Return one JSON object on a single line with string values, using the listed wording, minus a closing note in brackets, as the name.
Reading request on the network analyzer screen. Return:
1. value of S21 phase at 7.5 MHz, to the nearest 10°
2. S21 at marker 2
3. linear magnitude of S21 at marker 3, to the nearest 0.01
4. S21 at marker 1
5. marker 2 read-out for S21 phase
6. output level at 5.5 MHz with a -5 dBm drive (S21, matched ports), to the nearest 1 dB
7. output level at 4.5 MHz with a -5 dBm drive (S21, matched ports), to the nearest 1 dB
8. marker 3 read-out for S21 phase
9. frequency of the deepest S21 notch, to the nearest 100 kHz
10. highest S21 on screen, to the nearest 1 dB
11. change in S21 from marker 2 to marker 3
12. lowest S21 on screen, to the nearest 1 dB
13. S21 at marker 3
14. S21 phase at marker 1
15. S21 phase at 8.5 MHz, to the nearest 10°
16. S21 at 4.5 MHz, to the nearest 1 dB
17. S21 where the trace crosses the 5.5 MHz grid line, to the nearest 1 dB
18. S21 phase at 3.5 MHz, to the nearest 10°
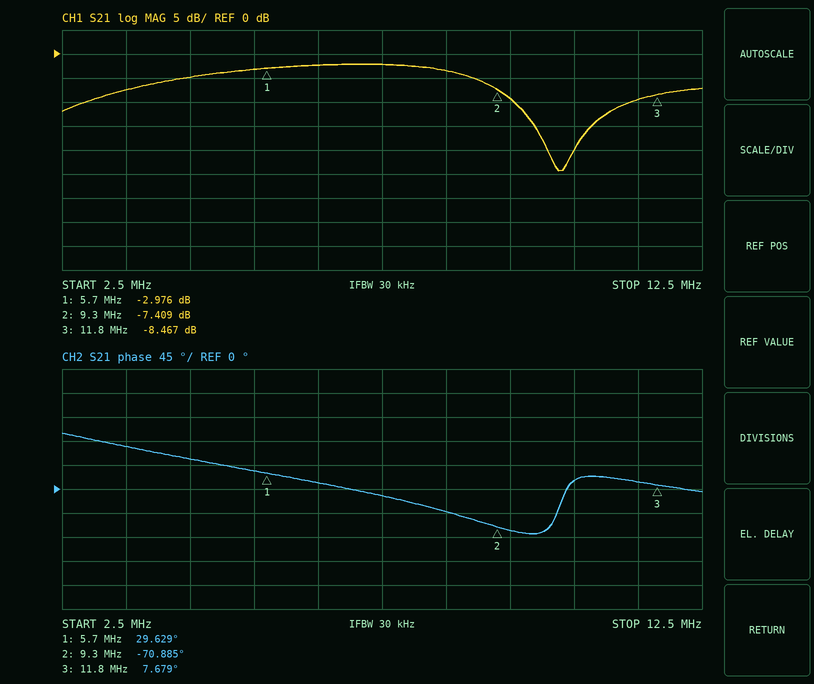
{"value of S21 phase at 7.5 MHz, to the nearest 10°": "-10°", "S21 at marker 2": "-7.409 dB", "linear magnitude of S21 at marker 3, to the nearest 0.01": "0.38", "S21 at marker 1": "-2.976 dB", "marker 2 read-out for S21 phase": "-70.885°", "output level at 5.5 MHz with a -5 dBm drive (S21, matched ports), to the nearest 1 dB": "-8 dBm", "output level at 4.5 MHz with a -5 dBm drive (S21, matched ports), to the nearest 1 dB": "-10 dBm", "marker 3 read-out for S21 phase": "7.679°", "frequency of the deepest S21 notch, to the nearest 100 kHz": "10.3 MHz", "highest S21 on screen, to the nearest 1 dB": "-2 dB", "change in S21 from marker 2 to marker 3": "-1.058 dB", "lowest S21 on screen, to the nearest 1 dB": "-24 dB", "S21 at marker 3": "-8.467 dB", "S21 phase at marker 1": "29.629°", "S21 phase at 8.5 MHz, to the nearest 10°": "-40°", "S21 at 4.5 MHz, to the nearest 1 dB": "-5 dB", "S21 where the trace crosses the 5.5 MHz grid line, to the nearest 1 dB": "-3 dB", "S21 phase at 3.5 MHz, to the nearest 10°": "80°"}
